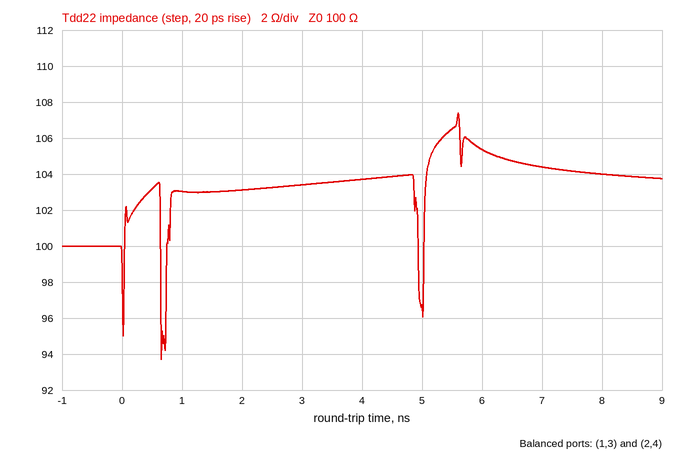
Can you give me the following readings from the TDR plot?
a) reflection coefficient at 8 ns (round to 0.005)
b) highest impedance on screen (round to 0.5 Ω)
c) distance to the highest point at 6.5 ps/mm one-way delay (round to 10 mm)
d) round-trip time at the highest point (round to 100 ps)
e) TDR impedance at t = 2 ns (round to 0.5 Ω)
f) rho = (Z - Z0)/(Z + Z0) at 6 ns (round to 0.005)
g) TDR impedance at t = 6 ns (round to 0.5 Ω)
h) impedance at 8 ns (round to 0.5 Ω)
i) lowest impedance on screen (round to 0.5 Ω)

+0.020
107.5 Ω
430 mm
5.6 ns
103.0 Ω
+0.025
105.5 Ω
104.0 Ω
93.5 Ω
